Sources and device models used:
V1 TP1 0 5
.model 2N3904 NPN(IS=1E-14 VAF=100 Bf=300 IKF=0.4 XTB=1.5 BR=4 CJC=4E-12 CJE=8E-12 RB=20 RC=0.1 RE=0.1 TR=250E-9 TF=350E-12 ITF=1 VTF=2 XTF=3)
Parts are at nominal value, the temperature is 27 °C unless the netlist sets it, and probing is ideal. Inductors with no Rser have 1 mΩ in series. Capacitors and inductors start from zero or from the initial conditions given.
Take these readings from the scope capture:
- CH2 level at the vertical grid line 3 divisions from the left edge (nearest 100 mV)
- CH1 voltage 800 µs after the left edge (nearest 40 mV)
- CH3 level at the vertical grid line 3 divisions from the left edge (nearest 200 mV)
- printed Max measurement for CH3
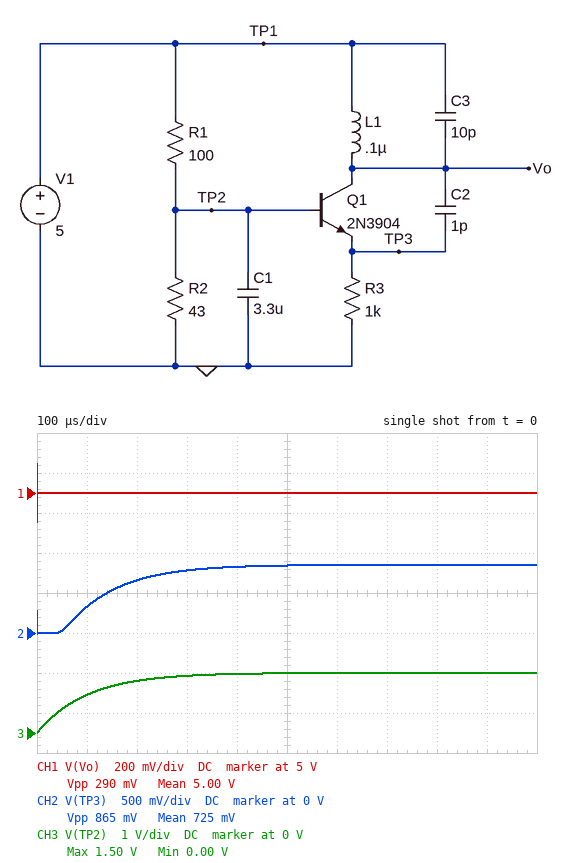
800 mV
5.00 V
1.4 V
1.50 V
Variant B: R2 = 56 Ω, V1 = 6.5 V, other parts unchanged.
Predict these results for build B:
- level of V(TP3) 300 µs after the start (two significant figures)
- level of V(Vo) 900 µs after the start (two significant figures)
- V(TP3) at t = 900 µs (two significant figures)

1.5 V
6.5 V
1.7 V
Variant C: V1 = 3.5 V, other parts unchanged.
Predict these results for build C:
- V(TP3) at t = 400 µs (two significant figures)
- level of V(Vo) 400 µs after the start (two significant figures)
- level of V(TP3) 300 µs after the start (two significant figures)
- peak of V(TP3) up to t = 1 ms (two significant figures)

400 mV
3.5 V
370 mV
420 mV
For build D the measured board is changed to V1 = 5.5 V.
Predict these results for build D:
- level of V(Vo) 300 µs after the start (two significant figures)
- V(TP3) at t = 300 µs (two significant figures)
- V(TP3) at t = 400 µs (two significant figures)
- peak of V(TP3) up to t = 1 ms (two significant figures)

5.5 V
920 mV
970 mV
1.0 V
